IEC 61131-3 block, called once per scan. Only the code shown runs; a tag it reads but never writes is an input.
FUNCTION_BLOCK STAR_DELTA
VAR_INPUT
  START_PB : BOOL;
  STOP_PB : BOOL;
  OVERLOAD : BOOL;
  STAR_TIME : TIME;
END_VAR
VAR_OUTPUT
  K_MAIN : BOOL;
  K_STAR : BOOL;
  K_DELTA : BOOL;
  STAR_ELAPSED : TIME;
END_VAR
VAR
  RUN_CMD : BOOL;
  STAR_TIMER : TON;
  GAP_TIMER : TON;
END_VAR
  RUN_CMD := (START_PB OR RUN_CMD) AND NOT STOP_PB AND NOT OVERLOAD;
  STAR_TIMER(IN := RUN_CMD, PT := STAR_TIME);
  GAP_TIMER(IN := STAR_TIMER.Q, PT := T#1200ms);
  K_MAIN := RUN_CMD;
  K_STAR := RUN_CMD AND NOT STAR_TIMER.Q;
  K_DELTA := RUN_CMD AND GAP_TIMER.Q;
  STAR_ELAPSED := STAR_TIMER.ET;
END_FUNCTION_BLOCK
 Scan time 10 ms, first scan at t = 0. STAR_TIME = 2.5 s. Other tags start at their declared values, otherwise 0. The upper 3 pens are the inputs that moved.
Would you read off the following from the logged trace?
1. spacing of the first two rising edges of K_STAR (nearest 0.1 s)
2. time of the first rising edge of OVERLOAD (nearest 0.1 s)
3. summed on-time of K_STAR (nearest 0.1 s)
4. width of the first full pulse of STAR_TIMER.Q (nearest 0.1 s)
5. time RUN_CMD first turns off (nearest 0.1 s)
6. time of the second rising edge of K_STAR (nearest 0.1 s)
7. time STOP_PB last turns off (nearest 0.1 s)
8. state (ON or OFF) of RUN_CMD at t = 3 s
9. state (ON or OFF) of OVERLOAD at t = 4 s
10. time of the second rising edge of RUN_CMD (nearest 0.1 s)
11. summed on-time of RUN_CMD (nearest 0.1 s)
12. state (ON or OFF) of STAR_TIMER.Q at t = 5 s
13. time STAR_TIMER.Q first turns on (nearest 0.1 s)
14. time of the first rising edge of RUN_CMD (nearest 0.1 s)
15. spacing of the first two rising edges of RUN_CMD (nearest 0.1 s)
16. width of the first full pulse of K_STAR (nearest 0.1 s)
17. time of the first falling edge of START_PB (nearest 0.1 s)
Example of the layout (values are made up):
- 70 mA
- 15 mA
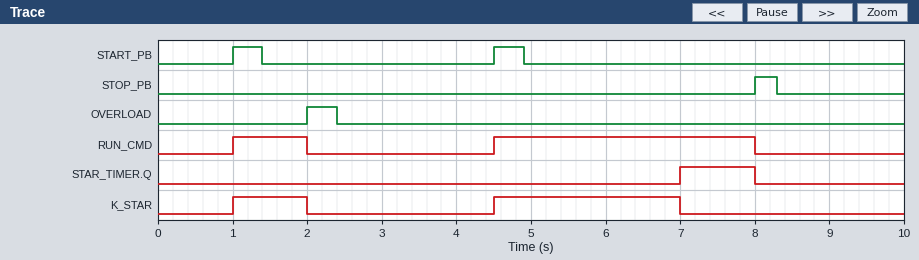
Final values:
- 3.5 s
- 2.0 s
- 3.5 s
- 1.0 s
- 2.0 s
- 4.5 s
- 8.3 s
- OFF
- OFF
- 4.5 s
- 4.5 s
- OFF
- 7.0 s
- 1.0 s
- 3.5 s
- 1.0 s
- 1.4 s
